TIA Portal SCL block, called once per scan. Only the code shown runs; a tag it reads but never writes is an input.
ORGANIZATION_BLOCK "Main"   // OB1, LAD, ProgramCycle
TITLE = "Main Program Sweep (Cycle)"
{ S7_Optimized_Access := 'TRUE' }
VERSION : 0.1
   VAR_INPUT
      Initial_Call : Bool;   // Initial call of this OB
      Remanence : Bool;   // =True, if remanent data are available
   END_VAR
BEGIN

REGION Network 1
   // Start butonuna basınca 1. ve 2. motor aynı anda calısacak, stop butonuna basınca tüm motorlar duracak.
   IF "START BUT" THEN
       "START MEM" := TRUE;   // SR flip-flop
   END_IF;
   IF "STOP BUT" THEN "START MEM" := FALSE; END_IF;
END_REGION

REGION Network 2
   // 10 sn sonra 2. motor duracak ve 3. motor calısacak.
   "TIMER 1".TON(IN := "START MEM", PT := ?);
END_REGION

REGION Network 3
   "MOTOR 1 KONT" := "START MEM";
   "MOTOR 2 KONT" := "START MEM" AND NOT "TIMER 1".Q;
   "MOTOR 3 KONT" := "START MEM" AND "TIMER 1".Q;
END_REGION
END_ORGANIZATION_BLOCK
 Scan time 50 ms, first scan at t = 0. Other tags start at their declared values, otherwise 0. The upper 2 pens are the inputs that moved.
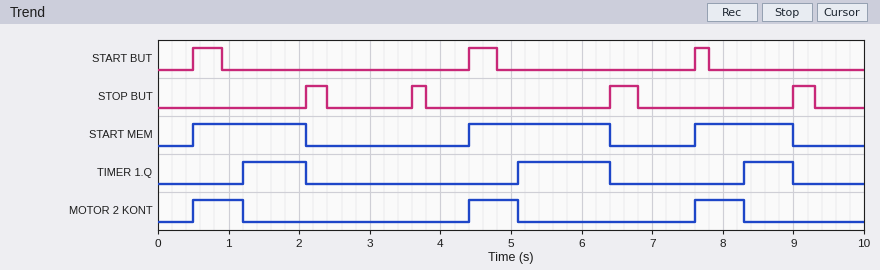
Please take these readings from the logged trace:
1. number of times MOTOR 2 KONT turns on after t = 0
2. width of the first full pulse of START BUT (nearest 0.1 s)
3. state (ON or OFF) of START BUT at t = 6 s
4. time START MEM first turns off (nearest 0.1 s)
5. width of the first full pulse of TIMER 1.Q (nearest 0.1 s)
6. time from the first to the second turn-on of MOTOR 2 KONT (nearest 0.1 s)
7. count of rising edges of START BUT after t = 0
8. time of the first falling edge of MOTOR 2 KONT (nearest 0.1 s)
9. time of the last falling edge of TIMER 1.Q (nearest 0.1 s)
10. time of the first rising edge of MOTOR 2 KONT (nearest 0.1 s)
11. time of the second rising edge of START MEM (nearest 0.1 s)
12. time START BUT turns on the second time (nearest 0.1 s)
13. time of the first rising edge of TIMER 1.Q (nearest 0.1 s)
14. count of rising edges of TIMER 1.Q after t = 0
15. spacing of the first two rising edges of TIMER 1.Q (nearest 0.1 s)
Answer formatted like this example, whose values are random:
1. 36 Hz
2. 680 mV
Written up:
1. 3
2. 0.4 s
3. OFF
4. 2.1 s
5. 0.9 s
6. 3.9 s
7. 3
8. 1.2 s
9. 9.0 s
10. 0.5 s
11. 4.4 s
12. 4.4 s
13. 1.2 s
14. 3
15. 3.9 s
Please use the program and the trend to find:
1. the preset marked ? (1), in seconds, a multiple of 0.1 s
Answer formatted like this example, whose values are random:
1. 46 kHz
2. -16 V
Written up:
1. 0.7 s
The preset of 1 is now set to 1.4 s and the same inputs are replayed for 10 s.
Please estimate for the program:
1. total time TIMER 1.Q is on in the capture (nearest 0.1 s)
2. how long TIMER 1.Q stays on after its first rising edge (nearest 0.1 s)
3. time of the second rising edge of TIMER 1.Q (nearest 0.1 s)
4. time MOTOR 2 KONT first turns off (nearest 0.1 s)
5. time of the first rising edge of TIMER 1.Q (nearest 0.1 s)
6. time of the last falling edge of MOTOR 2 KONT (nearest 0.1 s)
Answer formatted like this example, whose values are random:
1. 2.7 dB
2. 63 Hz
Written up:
1. 0.8 s
2. 0.2 s
3. 5.8 s
4. 1.9 s
5. 1.9 s
6. 9.0 s
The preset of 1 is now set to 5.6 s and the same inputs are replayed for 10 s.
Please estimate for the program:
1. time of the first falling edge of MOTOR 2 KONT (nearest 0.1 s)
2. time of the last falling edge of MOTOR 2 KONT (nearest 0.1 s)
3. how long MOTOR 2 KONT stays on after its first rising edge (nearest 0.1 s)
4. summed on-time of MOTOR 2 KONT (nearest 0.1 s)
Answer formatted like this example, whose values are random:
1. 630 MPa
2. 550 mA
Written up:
1. 2.1 s
2. 9.0 s
3. 1.6 s
4. 5.0 s
